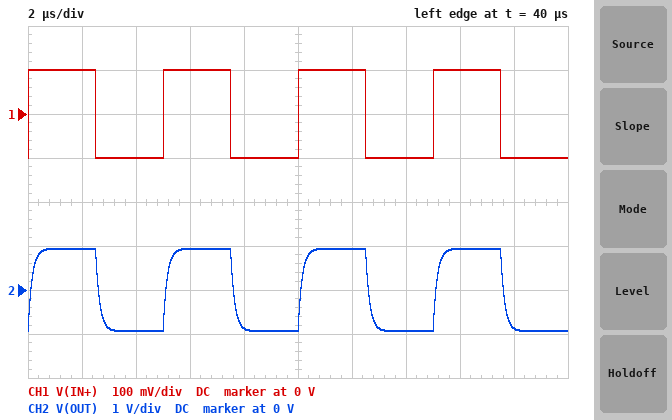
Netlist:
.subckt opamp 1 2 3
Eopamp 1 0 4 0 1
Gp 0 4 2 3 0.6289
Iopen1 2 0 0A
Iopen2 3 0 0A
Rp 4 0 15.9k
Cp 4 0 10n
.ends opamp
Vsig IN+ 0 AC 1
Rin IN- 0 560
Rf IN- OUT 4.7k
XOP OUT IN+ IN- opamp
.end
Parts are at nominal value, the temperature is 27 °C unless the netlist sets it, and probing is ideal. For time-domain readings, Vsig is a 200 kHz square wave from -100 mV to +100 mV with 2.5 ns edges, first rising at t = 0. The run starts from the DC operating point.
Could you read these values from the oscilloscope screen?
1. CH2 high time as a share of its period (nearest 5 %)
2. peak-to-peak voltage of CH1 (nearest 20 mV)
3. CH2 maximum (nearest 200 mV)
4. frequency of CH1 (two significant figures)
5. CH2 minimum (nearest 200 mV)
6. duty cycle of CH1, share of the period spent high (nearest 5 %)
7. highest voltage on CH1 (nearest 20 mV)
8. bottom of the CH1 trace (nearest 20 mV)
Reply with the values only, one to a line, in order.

50 %
200 mV
1.0 V
200 kHz
-1.0 V
50 %
100 mV
-100 mV
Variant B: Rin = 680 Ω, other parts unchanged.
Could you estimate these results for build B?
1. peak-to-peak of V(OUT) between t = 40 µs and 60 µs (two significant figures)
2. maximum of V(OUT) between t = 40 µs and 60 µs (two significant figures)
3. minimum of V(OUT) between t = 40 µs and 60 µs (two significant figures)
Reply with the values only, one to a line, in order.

1.6 V
790 mV
-790 mV
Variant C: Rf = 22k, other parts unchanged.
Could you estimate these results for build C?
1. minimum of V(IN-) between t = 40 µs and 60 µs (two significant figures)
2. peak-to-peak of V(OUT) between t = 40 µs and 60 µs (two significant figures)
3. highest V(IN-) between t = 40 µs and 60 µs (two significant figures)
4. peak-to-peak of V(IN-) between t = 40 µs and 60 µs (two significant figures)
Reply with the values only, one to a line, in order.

-96 mV
7.7 V
96 mV
190 mV
